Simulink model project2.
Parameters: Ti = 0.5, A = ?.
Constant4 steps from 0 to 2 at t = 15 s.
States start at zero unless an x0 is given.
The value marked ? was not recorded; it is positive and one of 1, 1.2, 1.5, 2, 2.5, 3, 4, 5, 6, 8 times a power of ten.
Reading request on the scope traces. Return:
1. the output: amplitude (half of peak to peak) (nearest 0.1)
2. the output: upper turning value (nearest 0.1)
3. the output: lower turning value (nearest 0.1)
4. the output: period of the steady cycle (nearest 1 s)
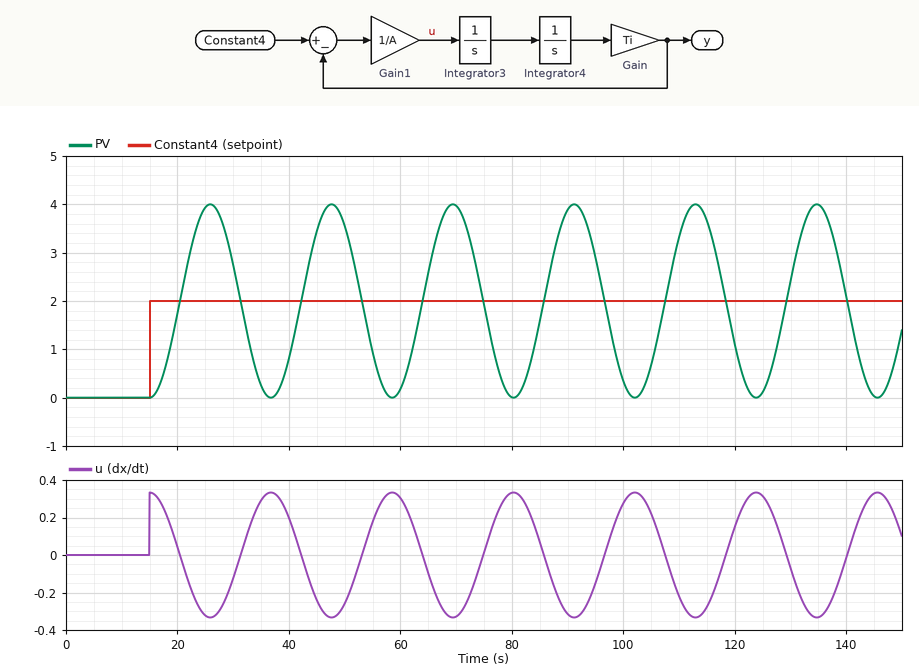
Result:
2.0
4.0
0.0
22 s
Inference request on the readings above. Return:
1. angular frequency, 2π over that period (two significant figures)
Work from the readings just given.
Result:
0.29 rad/s
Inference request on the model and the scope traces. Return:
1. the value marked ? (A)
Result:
6
